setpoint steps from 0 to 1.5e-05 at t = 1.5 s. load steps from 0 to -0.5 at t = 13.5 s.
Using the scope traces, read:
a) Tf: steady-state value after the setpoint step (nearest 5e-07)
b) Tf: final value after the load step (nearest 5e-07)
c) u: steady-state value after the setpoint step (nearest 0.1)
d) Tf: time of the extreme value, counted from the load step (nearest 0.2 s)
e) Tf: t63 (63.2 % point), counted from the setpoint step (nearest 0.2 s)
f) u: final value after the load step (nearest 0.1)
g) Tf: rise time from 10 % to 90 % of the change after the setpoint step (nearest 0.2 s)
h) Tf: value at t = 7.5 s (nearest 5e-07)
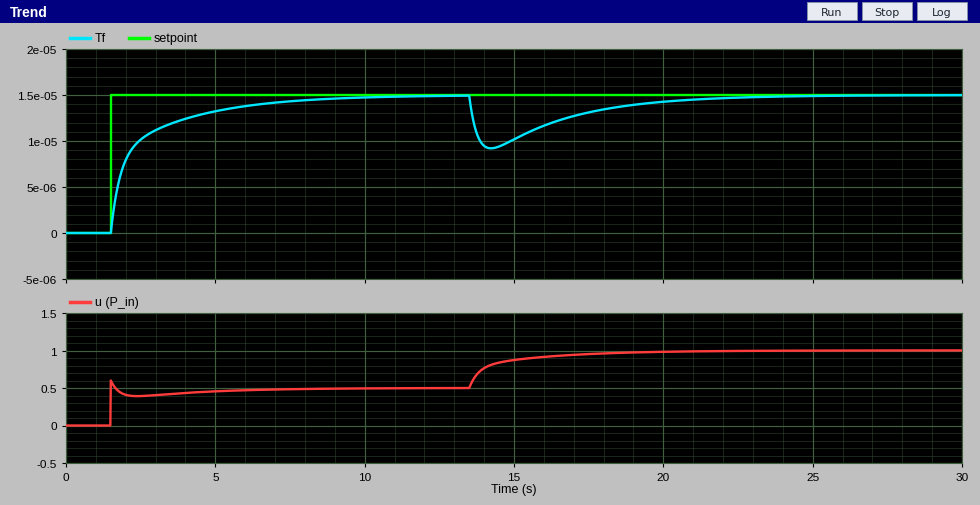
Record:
0.0000150
0.0000150
0.5
0.8 s
0.8 s
1.0
3.8 s
0.0000145
